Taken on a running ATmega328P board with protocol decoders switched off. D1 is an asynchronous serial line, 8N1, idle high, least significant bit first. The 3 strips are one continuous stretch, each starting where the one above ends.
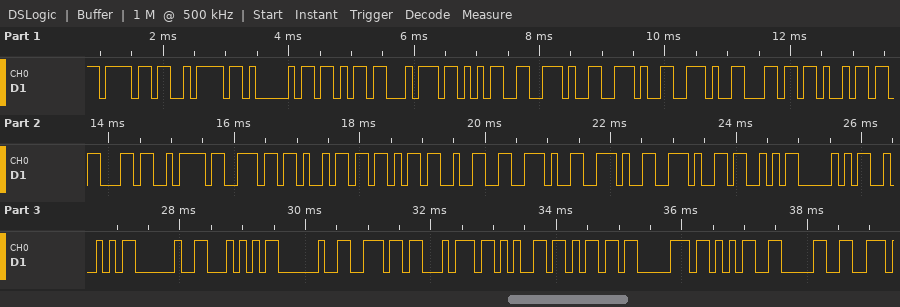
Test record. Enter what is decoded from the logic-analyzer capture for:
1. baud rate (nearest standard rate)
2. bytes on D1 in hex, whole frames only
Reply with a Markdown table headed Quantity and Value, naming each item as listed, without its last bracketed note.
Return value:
| Quantity | Value |
|---|---|
| baud rate | 9600 baud |
| bytes on D1 in hex, whole frames only | 0x6F 0x7A 0x41 0x6B 0x74 0x35 0x2E 0x2E 0x2E 0x6C 0x69 0x63 0x7A 0x6E 0x69 0x6B 0x32 0x2E 0x2E 0x2E 0x53 0x50 0x52 0x20 0x54 0x20 0x6E 0x74 0x65 0x6D 0x70 0x35 0x30 |
